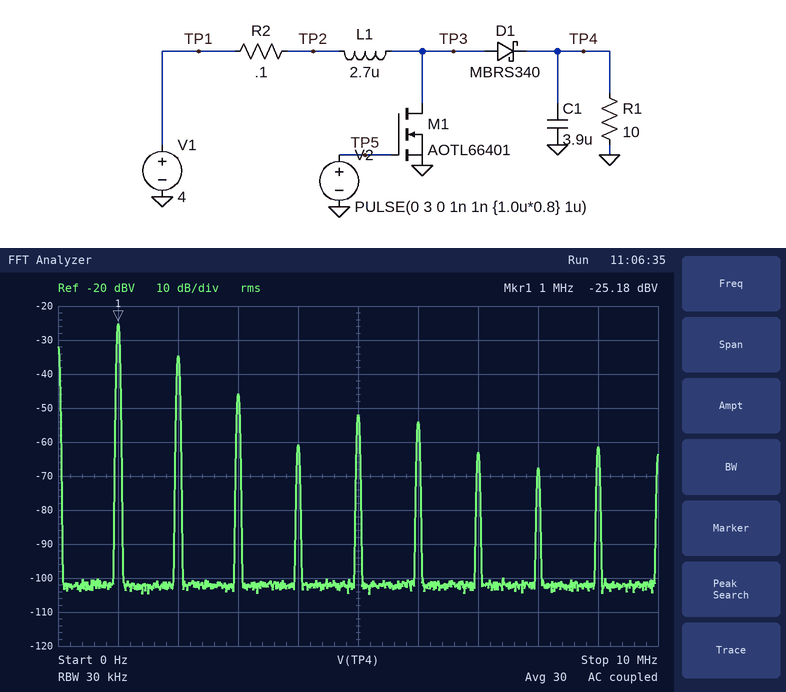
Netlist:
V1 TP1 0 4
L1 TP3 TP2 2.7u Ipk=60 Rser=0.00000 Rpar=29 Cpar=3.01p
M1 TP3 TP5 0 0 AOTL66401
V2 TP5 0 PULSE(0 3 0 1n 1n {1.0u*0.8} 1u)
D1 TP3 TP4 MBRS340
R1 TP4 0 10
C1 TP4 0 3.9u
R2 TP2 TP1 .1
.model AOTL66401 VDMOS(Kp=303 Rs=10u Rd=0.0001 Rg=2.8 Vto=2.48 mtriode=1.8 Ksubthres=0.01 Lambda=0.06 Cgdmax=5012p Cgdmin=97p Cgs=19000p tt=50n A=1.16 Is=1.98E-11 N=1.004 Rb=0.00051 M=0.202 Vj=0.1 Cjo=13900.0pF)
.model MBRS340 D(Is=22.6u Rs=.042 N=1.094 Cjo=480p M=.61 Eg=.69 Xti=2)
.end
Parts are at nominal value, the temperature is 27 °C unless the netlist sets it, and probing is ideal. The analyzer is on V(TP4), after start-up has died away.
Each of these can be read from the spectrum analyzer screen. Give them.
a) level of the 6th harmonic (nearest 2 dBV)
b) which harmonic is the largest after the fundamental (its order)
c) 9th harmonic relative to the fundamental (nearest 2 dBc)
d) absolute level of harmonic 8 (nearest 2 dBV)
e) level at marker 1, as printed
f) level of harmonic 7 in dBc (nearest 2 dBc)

-54 dBV
2
-36 dBc
-68 dBV
-25.18 dBV
-38 dBc
